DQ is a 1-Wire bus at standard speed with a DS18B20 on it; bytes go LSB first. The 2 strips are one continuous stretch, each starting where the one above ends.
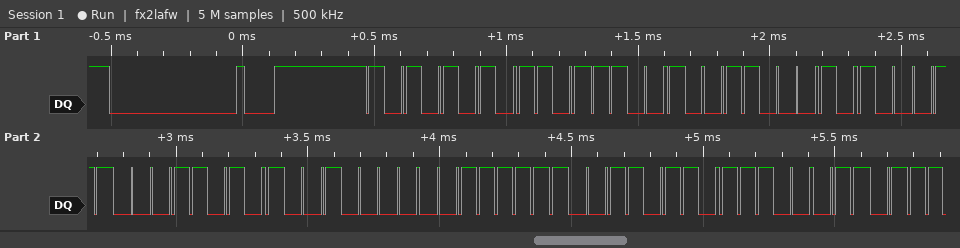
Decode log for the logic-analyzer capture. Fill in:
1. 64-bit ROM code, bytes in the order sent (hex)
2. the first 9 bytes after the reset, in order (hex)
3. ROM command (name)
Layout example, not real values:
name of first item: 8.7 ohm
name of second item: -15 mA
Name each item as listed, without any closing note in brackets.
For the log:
64-bit ROM code, bytes in the order sent: 3B 19 C5 58 09 FC 6C C7
the first 9 bytes after the reset, in order: 55 3B 19 C5 58 09 FC 6C C7
ROM command: Match ROM
